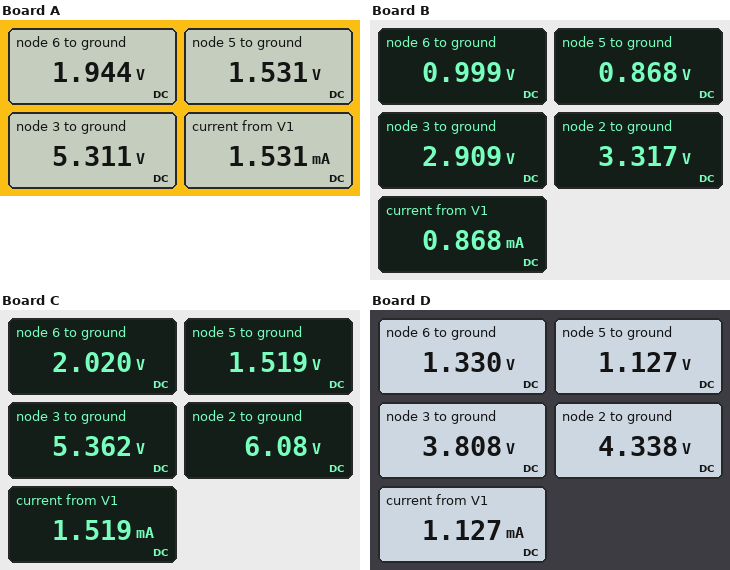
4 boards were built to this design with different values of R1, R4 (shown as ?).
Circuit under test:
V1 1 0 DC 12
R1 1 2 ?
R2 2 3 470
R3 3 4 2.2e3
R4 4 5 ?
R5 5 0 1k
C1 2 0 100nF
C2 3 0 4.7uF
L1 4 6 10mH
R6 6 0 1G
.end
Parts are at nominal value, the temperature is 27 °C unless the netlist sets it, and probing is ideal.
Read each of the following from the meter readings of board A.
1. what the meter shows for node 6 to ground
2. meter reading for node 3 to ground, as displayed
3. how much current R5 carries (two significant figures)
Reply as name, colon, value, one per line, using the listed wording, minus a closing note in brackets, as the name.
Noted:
what the meter shows for node 6 to ground: 1.944 V
meter reading for node 3 to ground, as displayed: 5.311 V
how much current R5 carries: 1.5 mA
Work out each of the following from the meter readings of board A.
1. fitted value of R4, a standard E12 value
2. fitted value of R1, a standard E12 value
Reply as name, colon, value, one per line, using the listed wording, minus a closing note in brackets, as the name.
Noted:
fitted value of R4, a standard E12 value: 270 Ω
fitted value of R1, a standard E12 value: 3.9 kΩ
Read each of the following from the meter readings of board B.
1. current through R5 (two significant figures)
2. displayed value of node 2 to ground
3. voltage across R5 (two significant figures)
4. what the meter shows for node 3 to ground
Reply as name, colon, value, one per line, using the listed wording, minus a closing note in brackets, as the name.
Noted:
current through R5: 870 µA
displayed value of node 2 to ground: 3.317 V
voltage across R5: 870 mV
what the meter shows for node 3 to ground: 2.909 V
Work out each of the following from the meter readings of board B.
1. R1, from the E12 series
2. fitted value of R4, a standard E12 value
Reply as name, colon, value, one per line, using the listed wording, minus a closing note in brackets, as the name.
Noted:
R1, from the E12 series: 10 kΩ
fitted value of R4, a standard E12 value: 150 Ω
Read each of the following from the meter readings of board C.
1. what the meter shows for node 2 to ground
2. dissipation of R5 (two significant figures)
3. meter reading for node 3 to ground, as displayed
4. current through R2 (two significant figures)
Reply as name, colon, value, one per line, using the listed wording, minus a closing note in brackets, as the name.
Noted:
what the meter shows for node 2 to ground: 6.08 V
dissipation of R5: 2.3 mW
meter reading for node 3 to ground, as displayed: 5.362 V
current through R2: 1.5 mA
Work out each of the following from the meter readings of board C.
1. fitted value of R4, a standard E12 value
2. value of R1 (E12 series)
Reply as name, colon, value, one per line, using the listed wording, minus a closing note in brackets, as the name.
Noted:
fitted value of R4, a standard E12 value: 330 Ω
value of R1: 3.9 kΩ
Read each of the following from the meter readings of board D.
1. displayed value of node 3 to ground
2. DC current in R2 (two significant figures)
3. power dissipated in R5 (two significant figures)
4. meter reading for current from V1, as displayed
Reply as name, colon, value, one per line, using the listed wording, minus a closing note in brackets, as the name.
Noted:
displayed value of node 3 to ground: 3.808 V
DC current in R2: 1.1 mA
power dissipated in R5: 1.3 mW
meter reading for current from V1, as displayed: 1.127 mA
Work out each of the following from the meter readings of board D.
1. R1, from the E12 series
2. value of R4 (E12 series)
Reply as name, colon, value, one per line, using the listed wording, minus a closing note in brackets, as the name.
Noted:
R1, from the E12 series: 6.8 kΩ
value of R4: 180 Ω
